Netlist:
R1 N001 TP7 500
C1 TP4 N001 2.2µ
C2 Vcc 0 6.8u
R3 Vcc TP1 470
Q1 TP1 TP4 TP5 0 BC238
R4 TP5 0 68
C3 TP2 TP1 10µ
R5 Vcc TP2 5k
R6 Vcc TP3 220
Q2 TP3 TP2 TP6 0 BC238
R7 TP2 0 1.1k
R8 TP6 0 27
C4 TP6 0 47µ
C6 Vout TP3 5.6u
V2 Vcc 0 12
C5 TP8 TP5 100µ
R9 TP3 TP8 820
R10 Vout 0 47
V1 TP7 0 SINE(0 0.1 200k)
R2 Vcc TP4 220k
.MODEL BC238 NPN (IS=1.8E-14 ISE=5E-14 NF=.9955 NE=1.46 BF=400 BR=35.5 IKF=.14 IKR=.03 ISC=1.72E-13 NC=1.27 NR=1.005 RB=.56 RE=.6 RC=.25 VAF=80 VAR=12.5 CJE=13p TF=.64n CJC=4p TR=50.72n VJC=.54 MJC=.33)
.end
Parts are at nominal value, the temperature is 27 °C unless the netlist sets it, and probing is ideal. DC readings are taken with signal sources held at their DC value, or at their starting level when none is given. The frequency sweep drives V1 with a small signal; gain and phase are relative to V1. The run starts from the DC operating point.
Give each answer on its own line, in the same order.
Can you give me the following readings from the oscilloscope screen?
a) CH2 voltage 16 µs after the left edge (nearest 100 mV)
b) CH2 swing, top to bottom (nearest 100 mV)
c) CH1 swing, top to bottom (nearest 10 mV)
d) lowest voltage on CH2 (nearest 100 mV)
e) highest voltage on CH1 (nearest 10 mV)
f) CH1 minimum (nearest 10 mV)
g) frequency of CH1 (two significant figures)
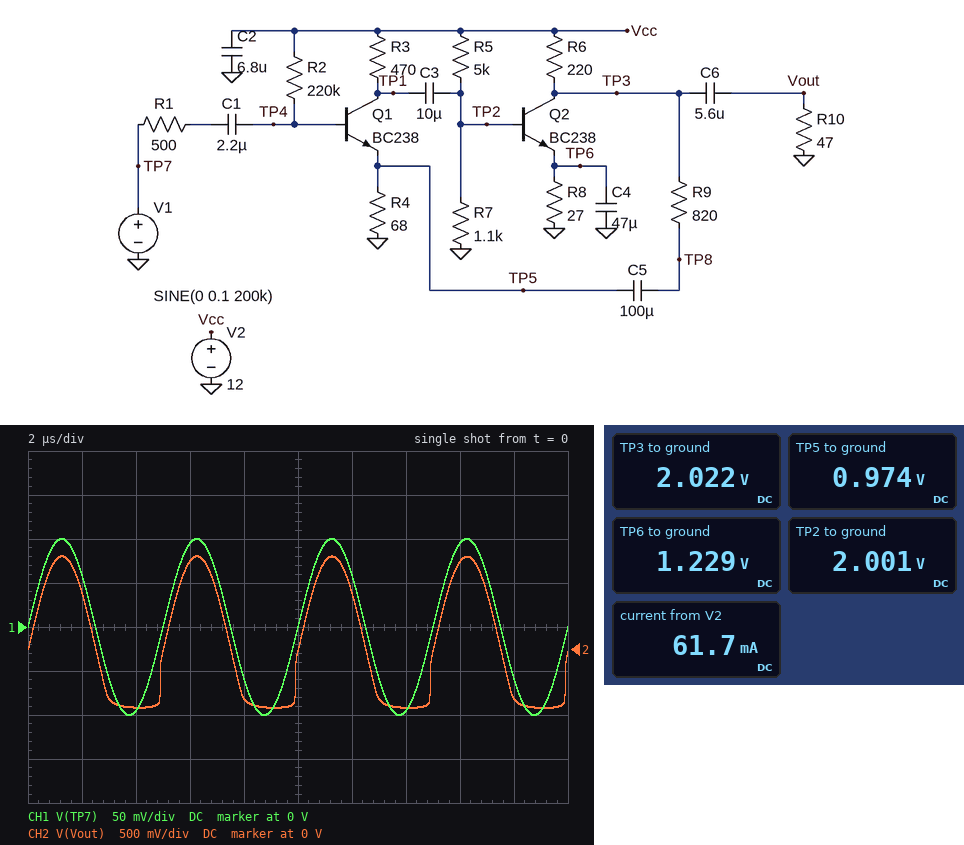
1.0 V
1.7 V
200 mV
-700 mV
100 mV
-100 mV
200 kHz
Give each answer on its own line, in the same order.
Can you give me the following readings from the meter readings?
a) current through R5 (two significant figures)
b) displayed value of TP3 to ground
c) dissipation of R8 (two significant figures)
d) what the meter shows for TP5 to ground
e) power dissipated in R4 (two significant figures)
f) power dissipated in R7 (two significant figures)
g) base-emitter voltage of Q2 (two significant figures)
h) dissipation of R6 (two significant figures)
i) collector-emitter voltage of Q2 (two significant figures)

2.0 mA
2.022 V
56 mW
0.974 V
14 mW
3.6 mW
770 mV
450 mW
790 mV
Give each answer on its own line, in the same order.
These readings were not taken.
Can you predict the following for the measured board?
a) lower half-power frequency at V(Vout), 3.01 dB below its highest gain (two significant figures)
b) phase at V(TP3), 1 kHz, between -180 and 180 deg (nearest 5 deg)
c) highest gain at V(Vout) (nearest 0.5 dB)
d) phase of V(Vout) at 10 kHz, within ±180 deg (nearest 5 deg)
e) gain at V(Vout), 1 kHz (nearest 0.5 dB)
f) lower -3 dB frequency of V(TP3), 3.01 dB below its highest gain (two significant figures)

730 Hz
5 deg
20.5 dB
5 deg
18.5 dB
4.2 Hz
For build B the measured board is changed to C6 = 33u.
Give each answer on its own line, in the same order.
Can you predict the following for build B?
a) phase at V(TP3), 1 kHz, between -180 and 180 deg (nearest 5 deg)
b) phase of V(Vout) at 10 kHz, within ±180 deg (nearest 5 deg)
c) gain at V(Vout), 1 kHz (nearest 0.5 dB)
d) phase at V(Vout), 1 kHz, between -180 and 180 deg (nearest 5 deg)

10 deg
0 deg
20.0 dB
15 deg
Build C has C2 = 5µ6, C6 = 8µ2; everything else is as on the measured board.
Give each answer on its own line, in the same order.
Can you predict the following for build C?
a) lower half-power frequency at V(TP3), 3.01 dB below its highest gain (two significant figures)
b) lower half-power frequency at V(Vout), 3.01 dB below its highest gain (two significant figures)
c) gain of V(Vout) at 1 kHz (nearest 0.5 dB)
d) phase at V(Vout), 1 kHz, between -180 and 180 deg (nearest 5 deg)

4.3 Hz
580 Hz
19.5 dB
30 deg
